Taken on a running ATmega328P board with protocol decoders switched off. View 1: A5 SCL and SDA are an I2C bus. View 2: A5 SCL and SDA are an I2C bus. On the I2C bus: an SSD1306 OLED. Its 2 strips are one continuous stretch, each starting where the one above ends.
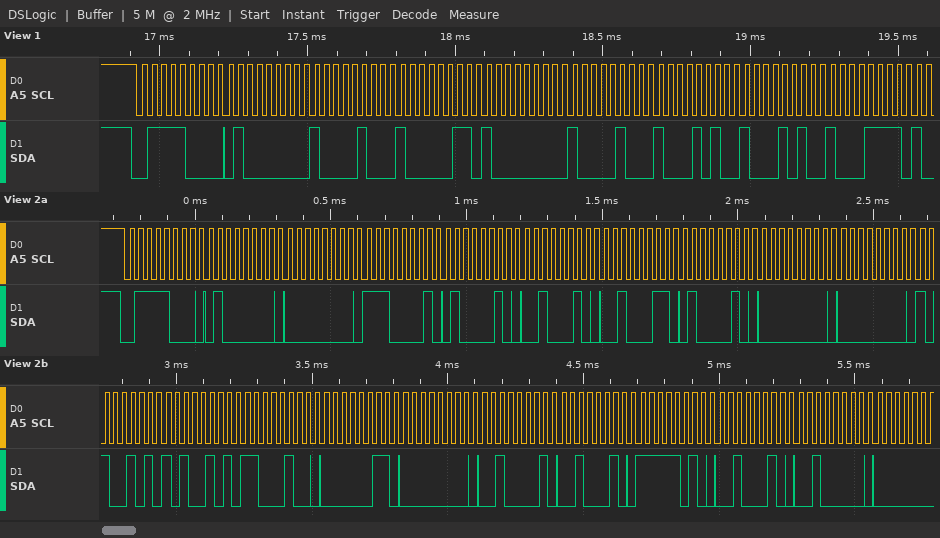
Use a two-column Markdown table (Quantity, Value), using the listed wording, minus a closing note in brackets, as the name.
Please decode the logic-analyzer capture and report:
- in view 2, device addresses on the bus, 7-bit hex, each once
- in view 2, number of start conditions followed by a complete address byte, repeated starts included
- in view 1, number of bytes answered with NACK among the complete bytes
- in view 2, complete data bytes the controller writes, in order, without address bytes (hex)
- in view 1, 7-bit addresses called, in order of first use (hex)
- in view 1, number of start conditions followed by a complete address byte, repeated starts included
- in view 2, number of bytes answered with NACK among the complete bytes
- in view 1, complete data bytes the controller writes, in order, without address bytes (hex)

| Quantity | Value |
|---|---|
| in view 2, device addresses on the bus, 7-bit hex, each once | 0x3C |
| in view 2, number of start conditions followed by a complete address byte, repeated starts included | 1 |
| in view 1, number of bytes answered with NACK among the complete bytes | 0 |
| in view 2, complete data bytes the controller writes, in order, without address bytes | 40 00 E1 42 22 23 42 00 00 A5 A5 C4 03 00 21 22 FA 22 20 |
| in view 1, 7-bit addresses called, in order of first use | 0x3C |
| in view 1, number of start conditions followed by a complete address byte, repeated starts included | 1 |
| in view 2, number of bytes answered with NACK among the complete bytes | 0 |
| in view 1, complete data bytes the controller writes, in order, without address bytes | 40 84 83 80 84 8A 8A 8F |
